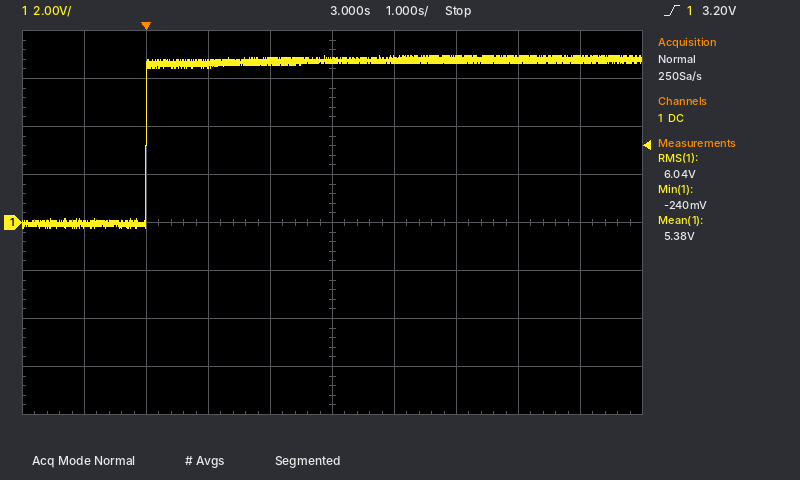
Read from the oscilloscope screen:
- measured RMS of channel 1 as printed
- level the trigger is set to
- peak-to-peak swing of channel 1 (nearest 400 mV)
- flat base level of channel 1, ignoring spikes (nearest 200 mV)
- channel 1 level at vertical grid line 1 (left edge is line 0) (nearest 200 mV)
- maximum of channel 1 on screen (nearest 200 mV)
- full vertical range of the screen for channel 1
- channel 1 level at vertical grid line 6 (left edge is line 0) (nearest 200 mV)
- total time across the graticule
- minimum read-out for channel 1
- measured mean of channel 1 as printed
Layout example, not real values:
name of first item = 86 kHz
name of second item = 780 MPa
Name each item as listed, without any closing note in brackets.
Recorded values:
measured RMS of channel 1 as printed = 6.04 V
level the trigger is set to = 3.20 V
peak-to-peak swing of channel 1 = 7.2 V
flat base level of channel 1, ignoring spikes = 0.0 V
channel 1 level at vertical grid line 1 (left edge is line 0) = 0.0 V
maximum of channel 1 on screen = 7.0 V
full vertical range of the screen for channel 1 = 16 V
channel 1 level at vertical grid line 6 (left edge is line 0) = 6.8 V
total time across the graticule = 10 s
minimum read-out for channel 1 = -240 mV
measured mean of channel 1 as printed = 5.38 V
